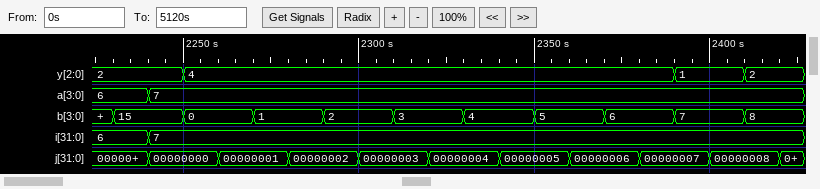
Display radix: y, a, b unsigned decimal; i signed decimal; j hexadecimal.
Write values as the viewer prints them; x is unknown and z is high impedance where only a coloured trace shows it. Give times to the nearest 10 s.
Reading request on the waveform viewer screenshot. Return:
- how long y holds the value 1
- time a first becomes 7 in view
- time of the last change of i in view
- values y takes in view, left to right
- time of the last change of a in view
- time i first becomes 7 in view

20 s
2240 s
2240 s
2, 4, 1, 2
2240 s
2240 s
